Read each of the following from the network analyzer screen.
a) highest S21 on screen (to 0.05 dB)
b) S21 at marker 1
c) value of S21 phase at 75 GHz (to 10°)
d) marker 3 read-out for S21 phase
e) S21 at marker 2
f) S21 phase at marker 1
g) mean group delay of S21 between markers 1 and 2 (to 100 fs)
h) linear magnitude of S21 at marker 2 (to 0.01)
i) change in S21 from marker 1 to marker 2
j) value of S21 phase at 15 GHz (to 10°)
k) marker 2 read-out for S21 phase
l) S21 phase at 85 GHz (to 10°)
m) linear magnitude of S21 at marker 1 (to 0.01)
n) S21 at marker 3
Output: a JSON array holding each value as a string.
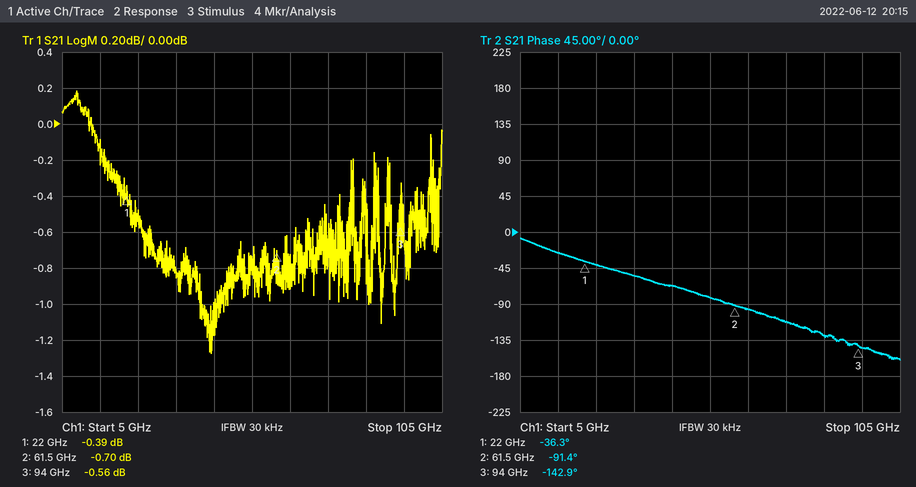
["0.20 dB", "-0.39 dB", "-110°", "-142.9°", "-0.70 dB", "-36.3°", "3.9 ps", "0.92", "-0.31 dB", "-30°", "-91.4°", "-130°", "0.96", "-0.56 dB"]
